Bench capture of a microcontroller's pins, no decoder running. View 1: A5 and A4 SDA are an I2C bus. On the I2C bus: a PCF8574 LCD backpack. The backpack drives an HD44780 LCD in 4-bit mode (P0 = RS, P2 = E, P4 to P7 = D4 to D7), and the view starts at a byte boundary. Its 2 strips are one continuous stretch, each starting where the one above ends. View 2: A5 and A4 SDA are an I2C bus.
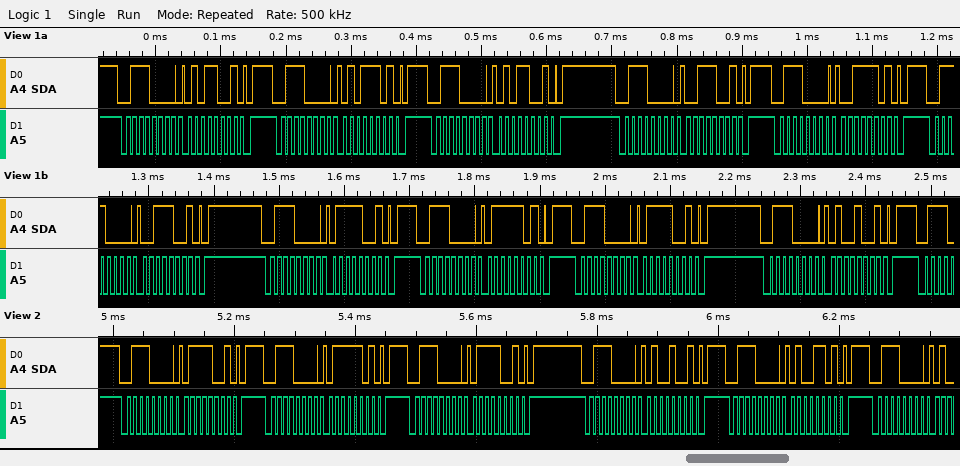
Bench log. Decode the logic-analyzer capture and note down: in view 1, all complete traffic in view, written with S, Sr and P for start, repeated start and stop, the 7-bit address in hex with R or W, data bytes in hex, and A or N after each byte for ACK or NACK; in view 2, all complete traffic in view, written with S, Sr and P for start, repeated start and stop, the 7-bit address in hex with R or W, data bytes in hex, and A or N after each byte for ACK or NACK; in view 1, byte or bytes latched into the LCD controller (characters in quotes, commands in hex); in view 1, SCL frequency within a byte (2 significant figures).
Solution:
S 38W A 59 A P S 38W A 5D A P S 38W A 59 A P S 38W A 39 A P S 38W A 3D A P S 38W A 39 A P S 38W A 79 A P S 38W A 7D A P S 38W A 79 A P S 38W A 49 A P
S 38W A 79 A P S 38W A 7D A P S 38W A 79 A P S 38W A 49 A P S 38W A 4D A P S 38W A
'S'
100 kHz
